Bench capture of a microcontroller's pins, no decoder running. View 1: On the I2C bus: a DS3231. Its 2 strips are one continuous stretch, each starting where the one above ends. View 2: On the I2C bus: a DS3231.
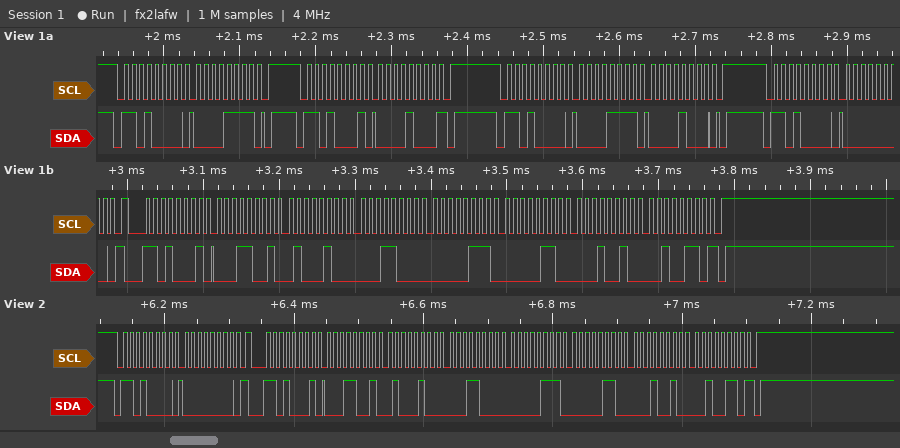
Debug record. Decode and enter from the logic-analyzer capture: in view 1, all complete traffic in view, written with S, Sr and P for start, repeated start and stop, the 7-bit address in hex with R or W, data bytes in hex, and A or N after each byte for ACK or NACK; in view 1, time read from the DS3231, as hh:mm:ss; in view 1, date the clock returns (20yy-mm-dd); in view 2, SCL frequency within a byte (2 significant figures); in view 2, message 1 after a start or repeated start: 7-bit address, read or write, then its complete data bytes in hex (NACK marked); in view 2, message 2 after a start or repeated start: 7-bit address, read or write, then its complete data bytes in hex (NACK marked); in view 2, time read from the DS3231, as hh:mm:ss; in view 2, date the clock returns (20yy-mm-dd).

S 68W A 0F A P S 68R A 08 N P S 68W A 0F A 08 A P S 68W A 00 A Sr 68R A 19 A 44 A 18 A 07 A 06 A 12 A 26 N P
18:44:19
2026-12-06
100 kHz
0x68 write: 00
0x68 read: 19 44 18 07 06 12 26 NACK
18:44:19
2026-12-06
